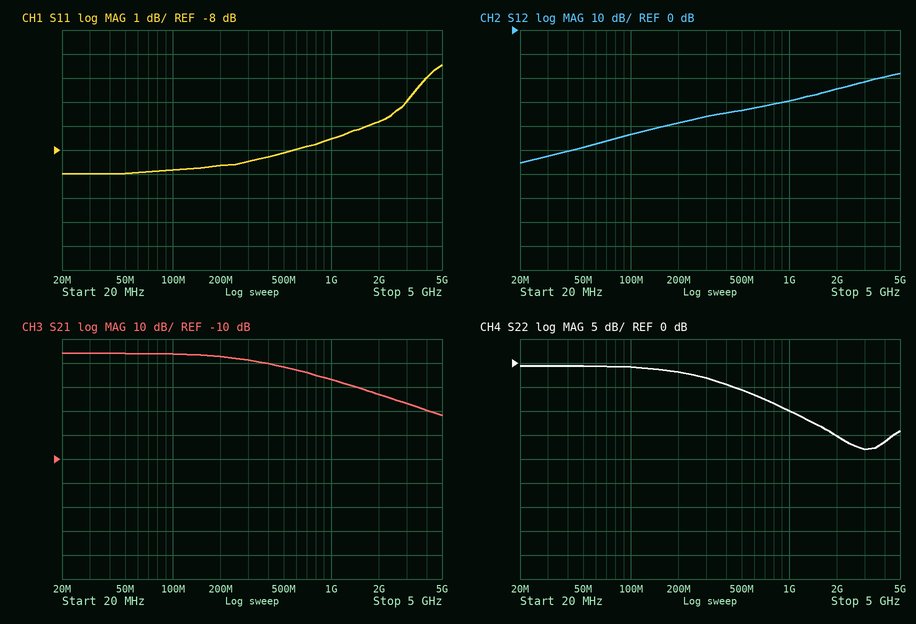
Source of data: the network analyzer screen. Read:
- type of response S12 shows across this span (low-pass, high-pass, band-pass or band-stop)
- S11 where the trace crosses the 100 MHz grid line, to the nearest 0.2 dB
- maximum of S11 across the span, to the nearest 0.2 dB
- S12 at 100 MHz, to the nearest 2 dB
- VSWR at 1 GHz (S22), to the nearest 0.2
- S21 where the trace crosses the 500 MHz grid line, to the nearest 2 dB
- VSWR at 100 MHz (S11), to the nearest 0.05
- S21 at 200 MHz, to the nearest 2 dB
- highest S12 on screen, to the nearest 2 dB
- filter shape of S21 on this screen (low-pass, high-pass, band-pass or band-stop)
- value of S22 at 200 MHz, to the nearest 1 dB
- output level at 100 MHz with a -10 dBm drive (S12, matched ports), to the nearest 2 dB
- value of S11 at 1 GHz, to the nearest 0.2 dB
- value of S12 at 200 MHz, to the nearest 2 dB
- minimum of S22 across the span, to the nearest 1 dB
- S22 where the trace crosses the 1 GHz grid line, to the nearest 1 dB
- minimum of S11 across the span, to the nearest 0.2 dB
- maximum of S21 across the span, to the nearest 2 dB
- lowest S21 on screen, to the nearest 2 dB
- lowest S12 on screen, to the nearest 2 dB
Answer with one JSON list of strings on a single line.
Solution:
["high-pass", "-8.8 dB", "-4.4 dB", "-44 dB", "2.0", "28 dB", "2.15", "32 dB", "-18 dB", "low-pass", "-2 dB", "-54 dBm", "-7.6 dB", "-38 dB", "-18 dB", "-10 dB", "-9.0 dB", "34 dB", "8 dB", "-56 dB"]
